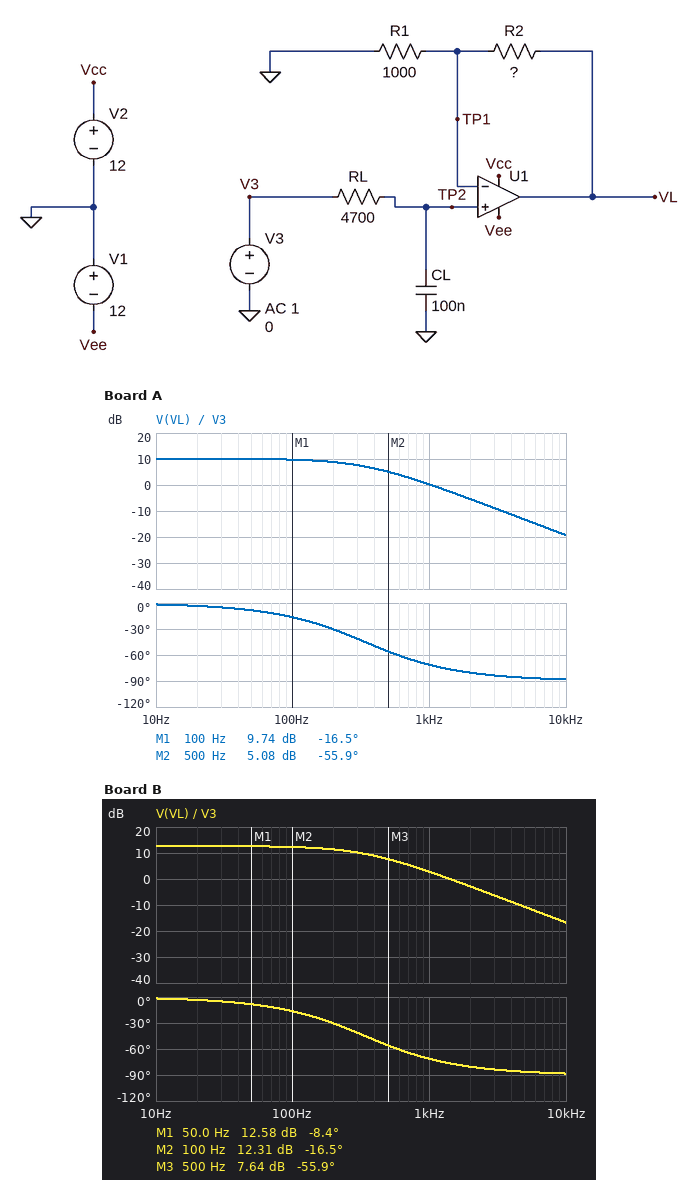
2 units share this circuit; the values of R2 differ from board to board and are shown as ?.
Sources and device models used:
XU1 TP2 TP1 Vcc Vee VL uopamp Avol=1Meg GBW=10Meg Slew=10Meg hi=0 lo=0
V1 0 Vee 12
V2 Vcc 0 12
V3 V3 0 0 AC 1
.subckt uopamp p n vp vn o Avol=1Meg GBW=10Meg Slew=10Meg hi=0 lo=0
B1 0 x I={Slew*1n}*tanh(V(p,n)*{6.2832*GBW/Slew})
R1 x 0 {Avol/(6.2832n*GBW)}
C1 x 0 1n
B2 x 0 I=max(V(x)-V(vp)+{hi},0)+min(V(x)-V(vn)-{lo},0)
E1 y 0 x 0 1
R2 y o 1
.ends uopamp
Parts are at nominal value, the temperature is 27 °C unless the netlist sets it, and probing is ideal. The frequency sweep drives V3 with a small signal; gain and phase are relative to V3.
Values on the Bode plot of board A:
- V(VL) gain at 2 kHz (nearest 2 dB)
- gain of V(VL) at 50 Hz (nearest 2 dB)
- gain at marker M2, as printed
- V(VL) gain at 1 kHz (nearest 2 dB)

-6 dB
10 dB
5.08 dB
0 dB
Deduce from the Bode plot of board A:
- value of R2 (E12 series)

2.2 kΩ
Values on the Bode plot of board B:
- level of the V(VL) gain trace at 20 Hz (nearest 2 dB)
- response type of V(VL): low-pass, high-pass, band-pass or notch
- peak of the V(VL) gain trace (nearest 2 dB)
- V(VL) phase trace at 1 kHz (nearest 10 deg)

12 dB
low-pass
12 dB
-70 deg
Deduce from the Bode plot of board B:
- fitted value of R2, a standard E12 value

3.3 kΩ
